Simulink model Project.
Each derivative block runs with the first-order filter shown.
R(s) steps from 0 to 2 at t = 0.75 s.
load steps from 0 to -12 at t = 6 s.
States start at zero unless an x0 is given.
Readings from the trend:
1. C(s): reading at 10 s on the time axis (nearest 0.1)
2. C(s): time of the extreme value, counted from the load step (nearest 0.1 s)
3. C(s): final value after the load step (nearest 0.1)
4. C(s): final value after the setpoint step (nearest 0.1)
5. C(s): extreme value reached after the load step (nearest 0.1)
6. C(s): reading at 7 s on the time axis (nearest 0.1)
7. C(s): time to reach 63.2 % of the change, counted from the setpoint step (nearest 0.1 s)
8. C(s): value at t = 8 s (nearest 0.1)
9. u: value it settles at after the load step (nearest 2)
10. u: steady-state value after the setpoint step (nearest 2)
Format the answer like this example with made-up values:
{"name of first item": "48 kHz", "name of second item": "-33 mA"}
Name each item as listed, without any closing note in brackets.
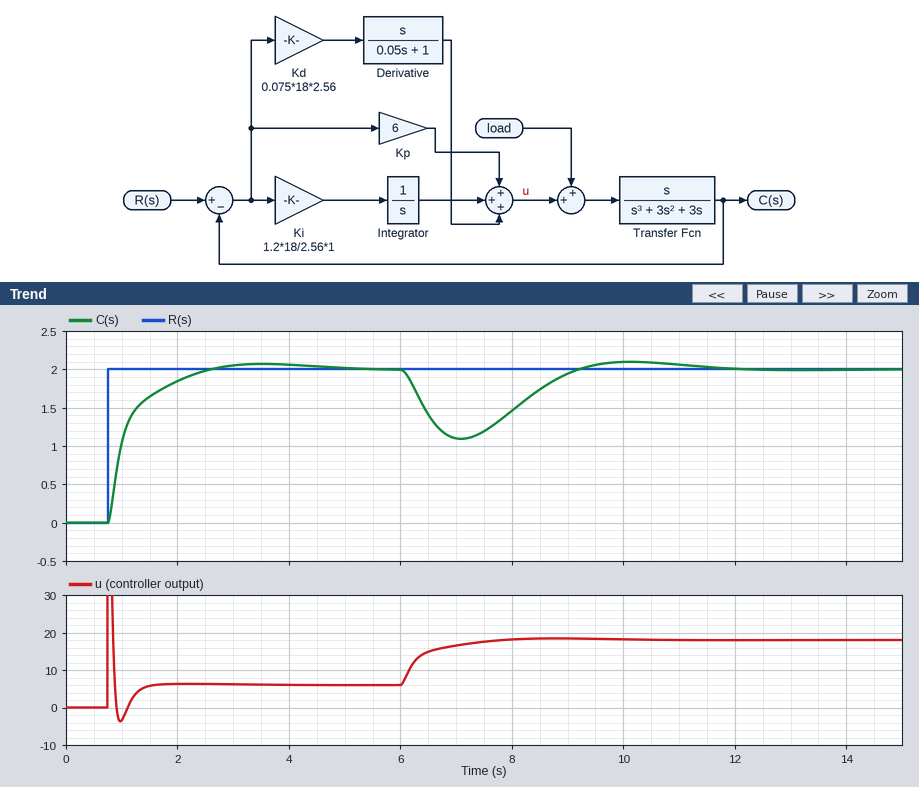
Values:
{"C(s): reading at 10 s on the time axis": "2.1", "C(s): time of the extreme value, counted from the load step": "1.1 s", "C(s): final value after the load step": "2.0", "C(s): final value after the setpoint step": "2.0", "C(s): extreme value reached after the load step": "1.1", "C(s): reading at 7 s on the time axis": "1.1", "C(s): time to reach 63.2 % of the change, counted from the setpoint step": "0.3 s", "C(s): value at t = 8 s": "1.5", "u: value it settles at after the load step": "18", "u: steady-state value after the setpoint step": "6"}
